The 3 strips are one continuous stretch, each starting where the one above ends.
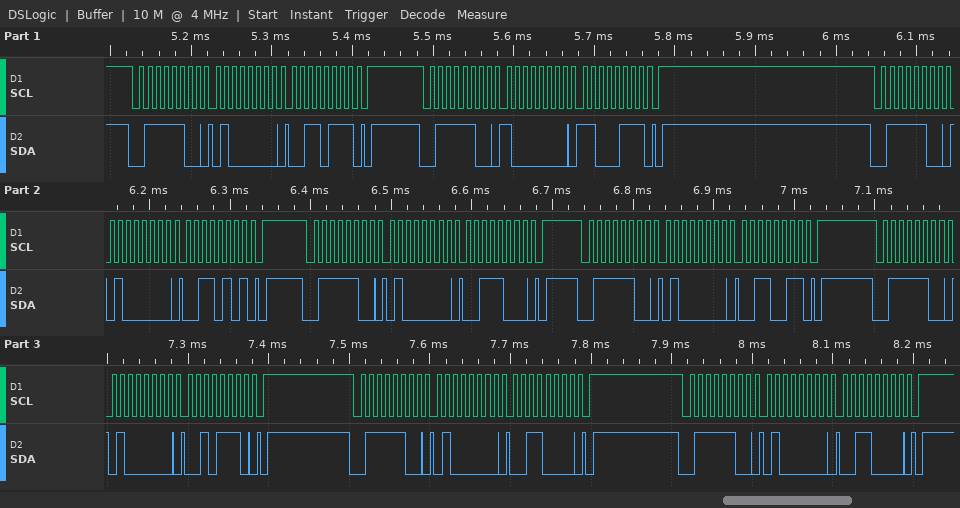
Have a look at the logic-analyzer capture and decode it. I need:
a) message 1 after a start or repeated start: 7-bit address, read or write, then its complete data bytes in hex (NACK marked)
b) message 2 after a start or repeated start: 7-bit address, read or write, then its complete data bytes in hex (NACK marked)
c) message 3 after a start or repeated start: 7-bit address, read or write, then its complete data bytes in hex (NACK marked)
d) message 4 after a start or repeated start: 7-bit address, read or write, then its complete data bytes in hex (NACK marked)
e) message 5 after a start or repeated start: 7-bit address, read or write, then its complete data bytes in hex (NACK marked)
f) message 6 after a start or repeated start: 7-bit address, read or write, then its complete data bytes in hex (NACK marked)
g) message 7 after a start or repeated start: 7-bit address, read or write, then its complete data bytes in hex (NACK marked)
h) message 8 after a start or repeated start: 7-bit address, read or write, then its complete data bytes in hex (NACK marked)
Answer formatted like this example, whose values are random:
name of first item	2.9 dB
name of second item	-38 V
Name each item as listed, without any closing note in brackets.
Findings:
message 1 after a start or repeated start: 7-bit address, read or write, then its complete data bytes in hex	0x3E write: 40 37
message 2 after a start or repeated start: 7-bit address, read or write, then its complete data bytes in hex	0x3E write: 80 C7
message 3 after a start or repeated start: 7-bit address, read or write, then its complete data bytes in hex	0x3E write: 40 35
message 4 after a start or repeated start: 7-bit address, read or write, then its complete data bytes in hex	0x3E write: 40 38
message 5 after a start or repeated start: 7-bit address, read or write, then its complete data bytes in hex	0x3E write: 40 33
message 6 after a start or repeated start: 7-bit address, read or write, then its complete data bytes in hex	0x3E write: 40 2E
message 7 after a start or repeated start: 7-bit address, read or write, then its complete data bytes in hex	0x3E write: 40 30
message 8 after a start or repeated start: 7-bit address, read or write, then its complete data bytes in hex	0x3E write: 40 30
